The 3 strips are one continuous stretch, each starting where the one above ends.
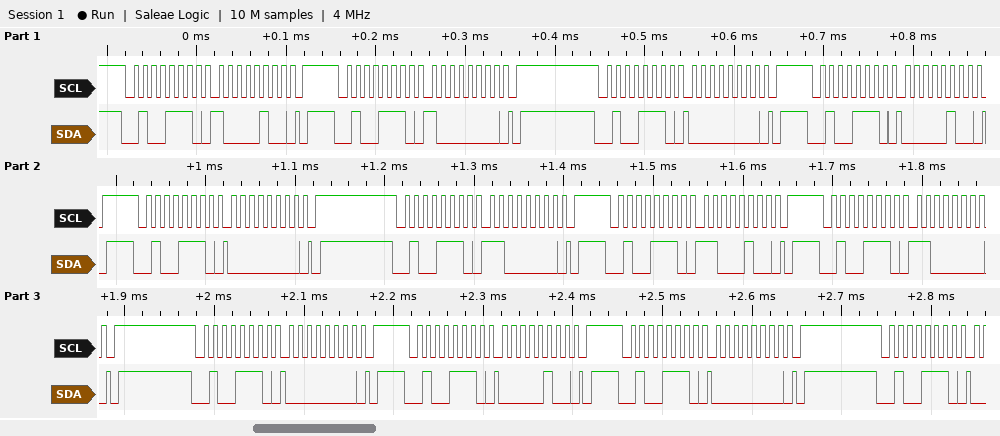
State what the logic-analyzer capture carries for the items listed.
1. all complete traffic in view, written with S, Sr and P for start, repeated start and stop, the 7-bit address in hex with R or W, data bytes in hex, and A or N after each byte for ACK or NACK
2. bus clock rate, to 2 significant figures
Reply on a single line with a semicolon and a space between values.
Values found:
S 27W A 84 A P S 27W A 80 A P S 27W A 00 A P S 27W A 04 A P S 27W A 00 A P S 27W A C0 A P S 27W A C4 A P S 27W A C0 A P S 27W A 00 A P S 27W A 04 A P S 27W A 00 A P S 27W A; 100 kHz
